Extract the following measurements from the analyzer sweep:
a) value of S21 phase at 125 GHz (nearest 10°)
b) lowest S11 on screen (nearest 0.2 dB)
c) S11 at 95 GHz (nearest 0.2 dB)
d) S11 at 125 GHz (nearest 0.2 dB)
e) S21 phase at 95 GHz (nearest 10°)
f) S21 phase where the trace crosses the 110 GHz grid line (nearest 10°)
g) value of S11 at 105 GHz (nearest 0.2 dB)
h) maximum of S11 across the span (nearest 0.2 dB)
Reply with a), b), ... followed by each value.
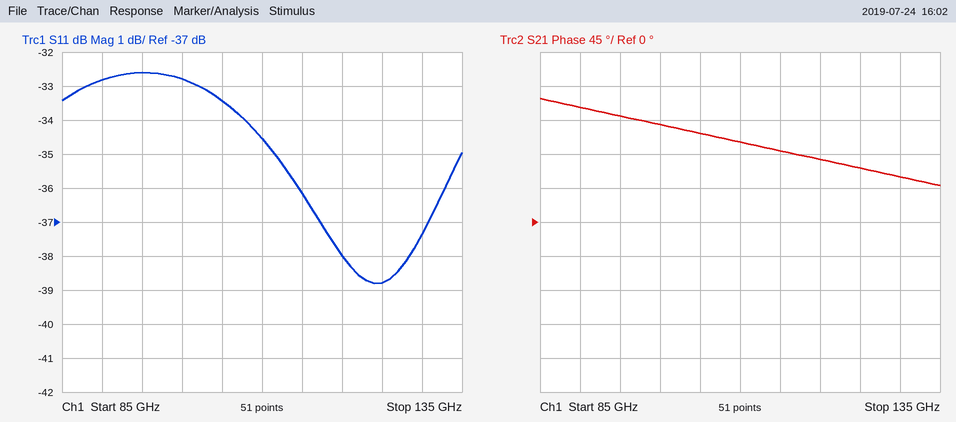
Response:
a) 70°
b) -38.8 dB
c) -32.6 dB
d) -38.8 dB
e) 140°
f) 110°
g) -33.4 dB
h) -32.6 dB
